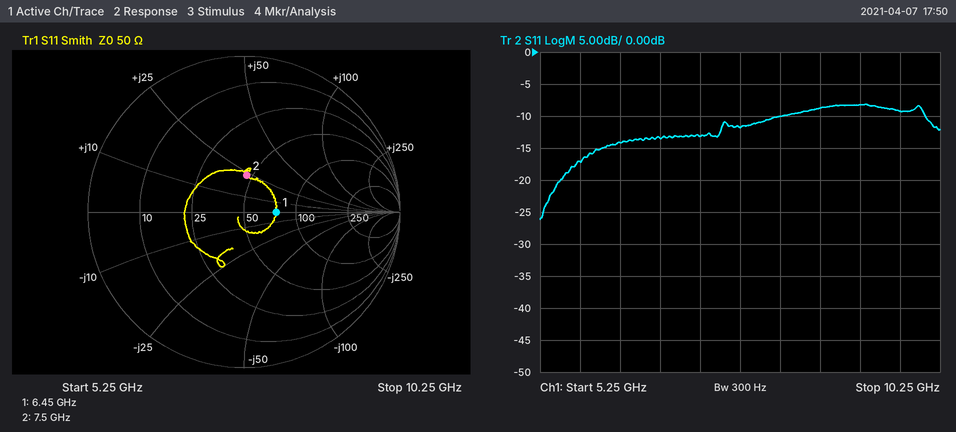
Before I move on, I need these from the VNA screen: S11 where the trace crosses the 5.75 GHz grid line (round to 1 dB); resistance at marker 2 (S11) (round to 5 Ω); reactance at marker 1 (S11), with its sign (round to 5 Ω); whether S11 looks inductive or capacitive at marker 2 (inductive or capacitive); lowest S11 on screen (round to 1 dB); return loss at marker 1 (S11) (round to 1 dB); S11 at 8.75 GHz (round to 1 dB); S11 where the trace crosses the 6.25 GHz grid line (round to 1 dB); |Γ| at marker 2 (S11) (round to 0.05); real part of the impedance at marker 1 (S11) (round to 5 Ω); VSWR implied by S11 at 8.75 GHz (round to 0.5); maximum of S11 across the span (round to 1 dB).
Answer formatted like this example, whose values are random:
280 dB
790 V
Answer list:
-17 dB
45 Ω
0 Ω
inductive
-26 dB
14 dB
-9 dB
-14 dB
0.25
75 Ω
2.0
-8 dB
